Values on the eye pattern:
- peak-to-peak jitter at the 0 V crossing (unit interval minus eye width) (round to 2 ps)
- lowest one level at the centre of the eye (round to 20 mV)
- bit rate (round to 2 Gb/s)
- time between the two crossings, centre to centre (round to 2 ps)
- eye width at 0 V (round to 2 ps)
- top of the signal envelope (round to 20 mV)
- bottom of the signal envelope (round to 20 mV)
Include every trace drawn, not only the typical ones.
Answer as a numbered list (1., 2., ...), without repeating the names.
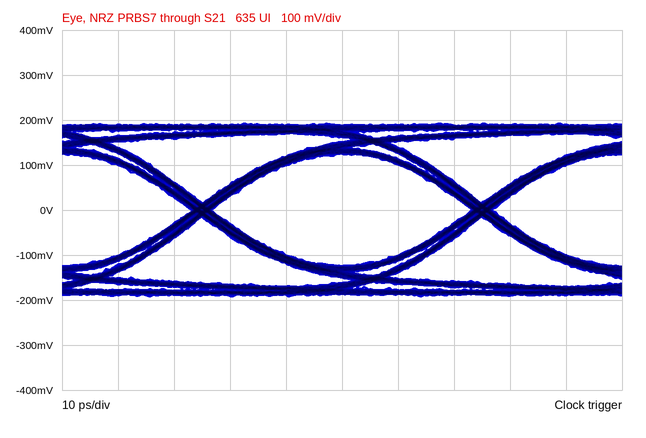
1. 4 ps
2. 120 mV
3. 20 Gb/s
4. 50 ps
5. 46 ps
6. 200 mV
7. -200 mV
